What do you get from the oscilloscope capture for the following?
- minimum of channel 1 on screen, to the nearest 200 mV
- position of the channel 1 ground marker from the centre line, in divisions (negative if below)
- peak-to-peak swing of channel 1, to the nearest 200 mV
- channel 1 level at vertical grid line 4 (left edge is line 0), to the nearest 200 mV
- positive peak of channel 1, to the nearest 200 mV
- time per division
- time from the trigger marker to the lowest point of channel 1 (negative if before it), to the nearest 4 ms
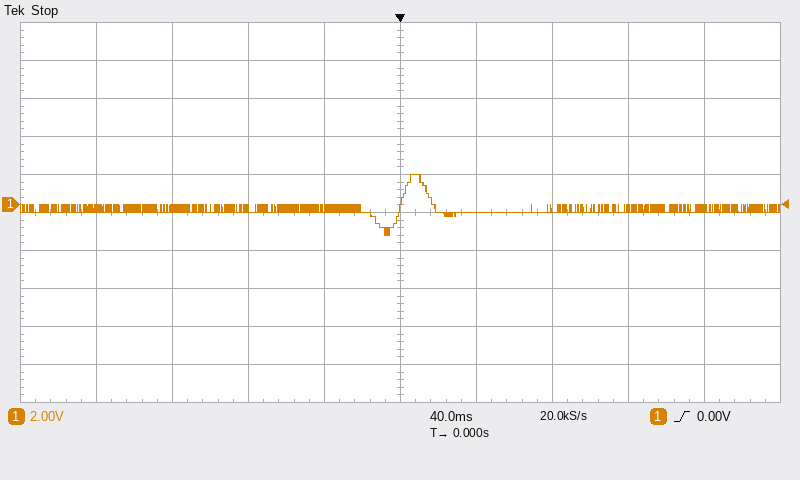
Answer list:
-1.6 V
+0.2 div
3.2 V
-200 mV
1.6 V
40 ms
-8 ms
